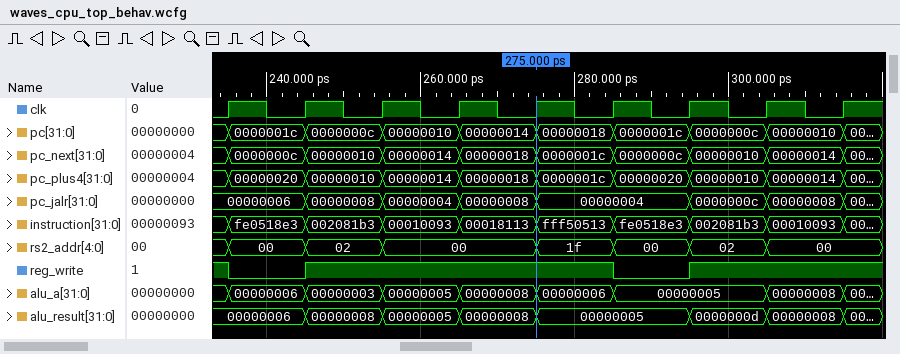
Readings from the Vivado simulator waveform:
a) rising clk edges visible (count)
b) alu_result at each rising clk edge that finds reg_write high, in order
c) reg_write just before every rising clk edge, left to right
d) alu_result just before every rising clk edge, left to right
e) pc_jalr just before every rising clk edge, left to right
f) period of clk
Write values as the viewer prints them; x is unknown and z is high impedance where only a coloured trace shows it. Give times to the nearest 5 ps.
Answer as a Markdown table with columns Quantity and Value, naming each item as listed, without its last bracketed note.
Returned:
| Quantity | Value |
|---|---|
| rising clk edges visible | 9 |
| alu_result at each rising clk edge that finds reg_write high, in order | 00000006, 00000008, 00000005, 00000008, 00000005, 0000000d, 00000008 |
| reg_write just before every rising clk edge, left to right | 1 0 1 1 1 1 0 1 1 |
| alu_result just before every rising clk edge, left to right | 00000006, 00000006, 00000008, 00000005, 00000008, 00000005, 00000005, 0000000d, 00000008 |
| pc_jalr just before every rising clk edge, left to right | 00000006, 00000006, 00000008, 00000004, 00000008, 00000004, 00000004, 0000000c, 00000008 |
| period of clk | 10 ps |
